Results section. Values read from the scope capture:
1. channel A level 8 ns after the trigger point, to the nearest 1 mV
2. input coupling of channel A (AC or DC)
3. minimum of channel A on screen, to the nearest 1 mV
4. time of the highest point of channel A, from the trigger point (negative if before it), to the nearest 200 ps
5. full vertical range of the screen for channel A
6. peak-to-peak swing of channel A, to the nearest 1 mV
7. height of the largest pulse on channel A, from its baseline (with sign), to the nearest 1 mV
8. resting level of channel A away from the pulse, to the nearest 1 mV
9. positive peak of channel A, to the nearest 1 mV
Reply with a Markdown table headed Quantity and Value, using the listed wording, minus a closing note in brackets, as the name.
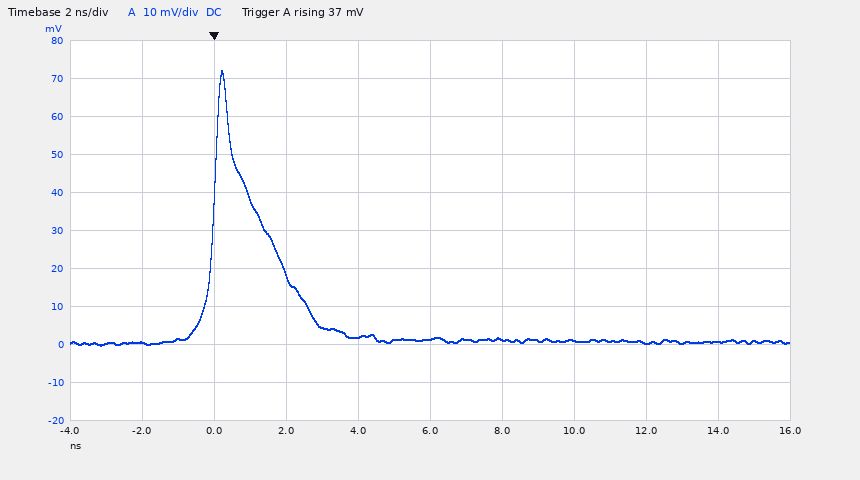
| Quantity | Value |
|---|---|
| channel A level 8 ns after the trigger point, to the nearest 1 mV | 1 mV |
| input coupling of channel A | DC |
| minimum of channel A on screen, to the nearest 1 mV | 0 mV |
| time of the highest point of channel A, from the trigger point (negative if before it), to the nearest 200 ps | +200 ps |
| full vertical range of the screen for channel A | 100 mV |
| peak-to-peak swing of channel A, to the nearest 1 mV | 72 mV |
| height of the largest pulse on channel A, from its baseline (with sign), to the nearest 1 mV | +71 mV |
| resting level of channel A away from the pulse, to the nearest 1 mV | 1 mV |
| positive peak of channel A, to the nearest 1 mV | 72 mV |
